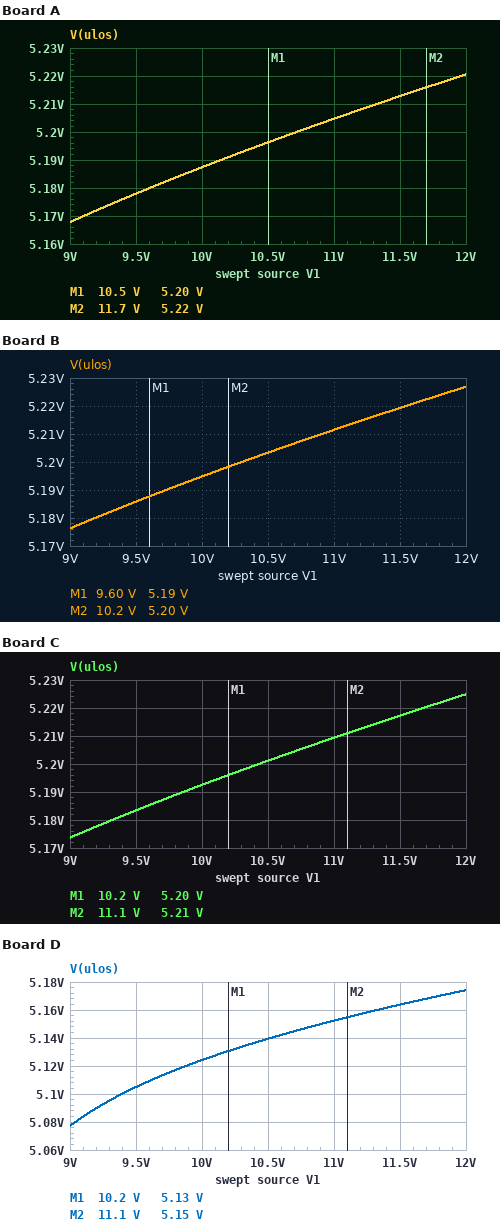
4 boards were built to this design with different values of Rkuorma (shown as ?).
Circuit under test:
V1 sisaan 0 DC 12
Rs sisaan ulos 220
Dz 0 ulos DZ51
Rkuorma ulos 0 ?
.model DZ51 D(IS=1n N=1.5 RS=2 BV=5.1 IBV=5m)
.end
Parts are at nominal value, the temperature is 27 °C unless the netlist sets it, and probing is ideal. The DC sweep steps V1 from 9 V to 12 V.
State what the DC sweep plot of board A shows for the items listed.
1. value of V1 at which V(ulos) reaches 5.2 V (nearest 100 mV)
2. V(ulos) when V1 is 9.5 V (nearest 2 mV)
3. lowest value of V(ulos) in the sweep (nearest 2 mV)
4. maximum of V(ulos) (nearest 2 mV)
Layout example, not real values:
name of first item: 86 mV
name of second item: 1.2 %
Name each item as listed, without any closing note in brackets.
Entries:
value of V1 at which V(ulos) reaches 5.2 V: 10.7 V
V(ulos) when V1 is 9.5 V: 5.178 V
lowest value of V(ulos) in the sweep: 5.168 V
maximum of V(ulos): 5.220 V
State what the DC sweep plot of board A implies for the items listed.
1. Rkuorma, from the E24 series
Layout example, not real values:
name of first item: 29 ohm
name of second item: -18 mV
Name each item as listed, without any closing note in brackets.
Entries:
Rkuorma, from the E24 series: 1.5 kΩ
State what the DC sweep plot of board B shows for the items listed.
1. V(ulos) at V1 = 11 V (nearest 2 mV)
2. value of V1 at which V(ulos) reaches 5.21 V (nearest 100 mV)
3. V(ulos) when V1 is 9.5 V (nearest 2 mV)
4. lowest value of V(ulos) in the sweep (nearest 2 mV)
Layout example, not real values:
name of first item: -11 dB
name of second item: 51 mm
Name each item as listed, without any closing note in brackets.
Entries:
V(ulos) at V1 = 11 V: 5.212 V
value of V1 at which V(ulos) reaches 5.21 V: 10.9 V
V(ulos) when V1 is 9.5 V: 5.186 V
lowest value of V(ulos) in the sweep: 5.176 V
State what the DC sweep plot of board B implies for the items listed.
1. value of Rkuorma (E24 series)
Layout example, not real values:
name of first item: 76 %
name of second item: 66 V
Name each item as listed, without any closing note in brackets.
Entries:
value of Rkuorma: 3.3 kΩ
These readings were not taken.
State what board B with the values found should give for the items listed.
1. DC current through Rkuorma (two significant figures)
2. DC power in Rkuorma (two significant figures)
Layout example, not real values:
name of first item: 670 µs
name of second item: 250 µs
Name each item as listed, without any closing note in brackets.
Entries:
DC current through Rkuorma: 1.6 mA
DC power in Rkuorma: 8.3 mW
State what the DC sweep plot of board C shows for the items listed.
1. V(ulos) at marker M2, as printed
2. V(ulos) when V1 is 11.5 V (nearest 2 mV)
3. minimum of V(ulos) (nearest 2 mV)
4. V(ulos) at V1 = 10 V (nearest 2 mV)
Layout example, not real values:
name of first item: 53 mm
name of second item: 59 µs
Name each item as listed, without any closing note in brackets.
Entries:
V(ulos) at marker M2, as printed: 5.21 V
V(ulos) when V1 is 11.5 V: 5.218 V
minimum of V(ulos): 5.174 V
V(ulos) at V1 = 10 V: 5.192 V
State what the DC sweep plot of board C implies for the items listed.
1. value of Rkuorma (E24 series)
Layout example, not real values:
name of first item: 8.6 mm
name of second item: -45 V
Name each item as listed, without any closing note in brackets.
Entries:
value of Rkuorma: 2.4 kΩ
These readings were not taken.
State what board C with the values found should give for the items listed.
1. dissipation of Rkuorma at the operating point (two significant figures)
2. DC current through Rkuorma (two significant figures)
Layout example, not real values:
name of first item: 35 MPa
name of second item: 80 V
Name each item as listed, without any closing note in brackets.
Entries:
dissipation of Rkuorma at the operating point: 11 mW
DC current through Rkuorma: 2.2 mA
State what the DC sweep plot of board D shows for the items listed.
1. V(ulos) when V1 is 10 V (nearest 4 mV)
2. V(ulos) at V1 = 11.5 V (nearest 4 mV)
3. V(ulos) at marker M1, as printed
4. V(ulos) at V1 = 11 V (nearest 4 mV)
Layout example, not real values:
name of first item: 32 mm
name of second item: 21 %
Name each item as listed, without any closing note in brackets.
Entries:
V(ulos) when V1 is 10 V: 5.124 V
V(ulos) at V1 = 11.5 V: 5.164 V
V(ulos) at marker M1, as printed: 5.13 V
V(ulos) at V1 = 11 V: 5.152 V
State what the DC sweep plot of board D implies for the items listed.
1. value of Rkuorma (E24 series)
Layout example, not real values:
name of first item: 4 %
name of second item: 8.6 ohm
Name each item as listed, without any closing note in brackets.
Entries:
value of Rkuorma: 330 Ω
